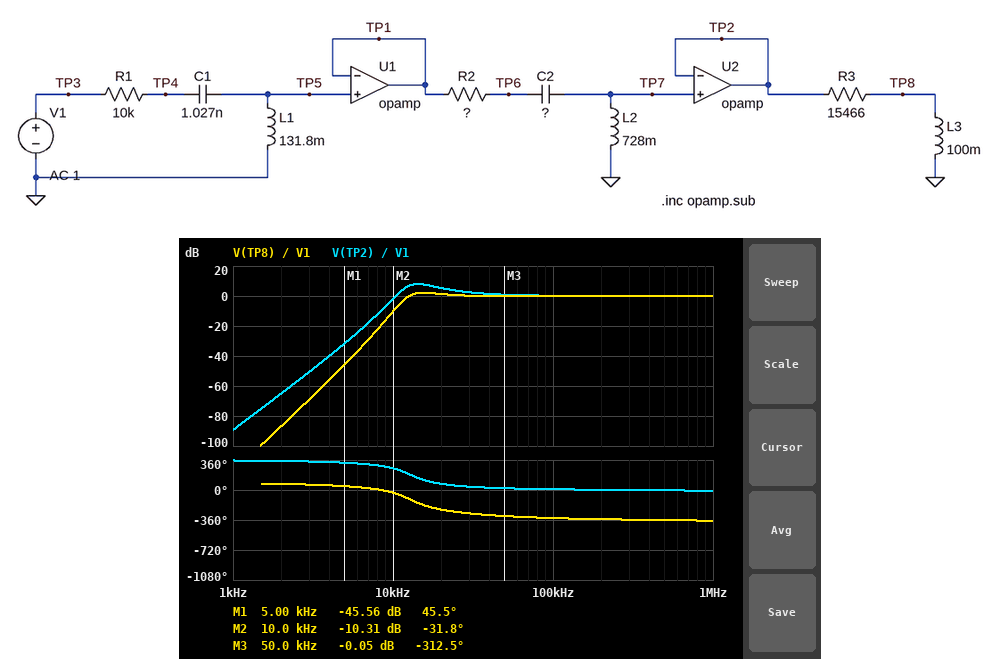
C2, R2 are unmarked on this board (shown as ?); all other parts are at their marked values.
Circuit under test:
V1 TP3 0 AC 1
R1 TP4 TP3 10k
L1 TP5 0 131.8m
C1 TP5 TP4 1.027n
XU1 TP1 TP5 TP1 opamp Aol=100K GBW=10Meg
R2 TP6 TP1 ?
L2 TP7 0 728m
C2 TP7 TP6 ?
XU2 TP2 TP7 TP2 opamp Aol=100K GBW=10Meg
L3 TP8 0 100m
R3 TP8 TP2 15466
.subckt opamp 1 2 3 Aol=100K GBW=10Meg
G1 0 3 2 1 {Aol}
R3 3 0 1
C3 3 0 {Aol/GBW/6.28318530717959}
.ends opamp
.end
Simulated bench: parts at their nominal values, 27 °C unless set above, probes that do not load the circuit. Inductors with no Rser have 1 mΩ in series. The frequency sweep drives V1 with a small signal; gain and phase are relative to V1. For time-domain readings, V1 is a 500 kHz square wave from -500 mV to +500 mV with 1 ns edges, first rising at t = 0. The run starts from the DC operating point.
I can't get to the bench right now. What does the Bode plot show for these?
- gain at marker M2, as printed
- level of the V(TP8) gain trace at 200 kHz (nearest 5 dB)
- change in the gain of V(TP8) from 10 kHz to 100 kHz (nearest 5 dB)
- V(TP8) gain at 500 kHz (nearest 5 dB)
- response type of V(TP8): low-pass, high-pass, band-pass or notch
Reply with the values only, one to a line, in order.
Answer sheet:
-10.31 dB
0 dB
10 dB
0 dB
high-pass
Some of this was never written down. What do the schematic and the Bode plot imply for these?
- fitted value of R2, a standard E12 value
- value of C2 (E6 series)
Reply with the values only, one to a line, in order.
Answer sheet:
27 kΩ
220 pF
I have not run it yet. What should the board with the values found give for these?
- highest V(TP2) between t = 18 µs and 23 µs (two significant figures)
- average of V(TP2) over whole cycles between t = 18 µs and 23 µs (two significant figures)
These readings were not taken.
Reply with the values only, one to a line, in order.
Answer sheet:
240 mV
-290 mV
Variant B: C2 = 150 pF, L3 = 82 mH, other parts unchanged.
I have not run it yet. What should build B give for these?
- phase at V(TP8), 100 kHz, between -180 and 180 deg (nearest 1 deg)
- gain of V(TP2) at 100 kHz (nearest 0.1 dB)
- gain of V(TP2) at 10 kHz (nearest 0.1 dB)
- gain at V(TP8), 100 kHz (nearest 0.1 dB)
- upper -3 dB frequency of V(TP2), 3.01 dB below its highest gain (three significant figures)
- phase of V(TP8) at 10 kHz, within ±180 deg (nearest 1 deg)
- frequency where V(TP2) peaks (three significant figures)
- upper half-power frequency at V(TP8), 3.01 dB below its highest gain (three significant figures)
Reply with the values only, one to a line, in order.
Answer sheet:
26 deg
0.3 dB
-6.7 dB
-0.1 dB
20.5 kHz
-7 deg
16.0 kHz
25.6 kHz
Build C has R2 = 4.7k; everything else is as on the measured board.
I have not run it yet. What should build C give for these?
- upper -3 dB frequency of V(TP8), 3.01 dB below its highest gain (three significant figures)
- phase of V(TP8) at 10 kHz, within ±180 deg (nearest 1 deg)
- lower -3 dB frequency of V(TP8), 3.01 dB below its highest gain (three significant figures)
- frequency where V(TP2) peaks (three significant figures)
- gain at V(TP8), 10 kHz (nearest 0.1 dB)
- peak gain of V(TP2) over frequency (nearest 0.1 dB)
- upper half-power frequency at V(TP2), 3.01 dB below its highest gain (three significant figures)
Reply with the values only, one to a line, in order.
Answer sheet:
13.3 kHz
4 deg
12.2 kHz
12.6 kHz
-7.4 dB
22.0 dB
13.2 kHz
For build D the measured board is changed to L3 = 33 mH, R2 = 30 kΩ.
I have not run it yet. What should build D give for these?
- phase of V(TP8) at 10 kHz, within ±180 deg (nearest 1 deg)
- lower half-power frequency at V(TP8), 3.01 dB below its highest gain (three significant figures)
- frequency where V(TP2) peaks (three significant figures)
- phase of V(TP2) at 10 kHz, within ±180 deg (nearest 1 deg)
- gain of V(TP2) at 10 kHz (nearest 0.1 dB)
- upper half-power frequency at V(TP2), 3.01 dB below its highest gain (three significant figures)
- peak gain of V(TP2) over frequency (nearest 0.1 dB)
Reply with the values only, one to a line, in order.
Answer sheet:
-20 deg
65.6 kHz
14.6 kHz
-103 deg
-2.3 dB
22.3 kHz
7.3 dB
